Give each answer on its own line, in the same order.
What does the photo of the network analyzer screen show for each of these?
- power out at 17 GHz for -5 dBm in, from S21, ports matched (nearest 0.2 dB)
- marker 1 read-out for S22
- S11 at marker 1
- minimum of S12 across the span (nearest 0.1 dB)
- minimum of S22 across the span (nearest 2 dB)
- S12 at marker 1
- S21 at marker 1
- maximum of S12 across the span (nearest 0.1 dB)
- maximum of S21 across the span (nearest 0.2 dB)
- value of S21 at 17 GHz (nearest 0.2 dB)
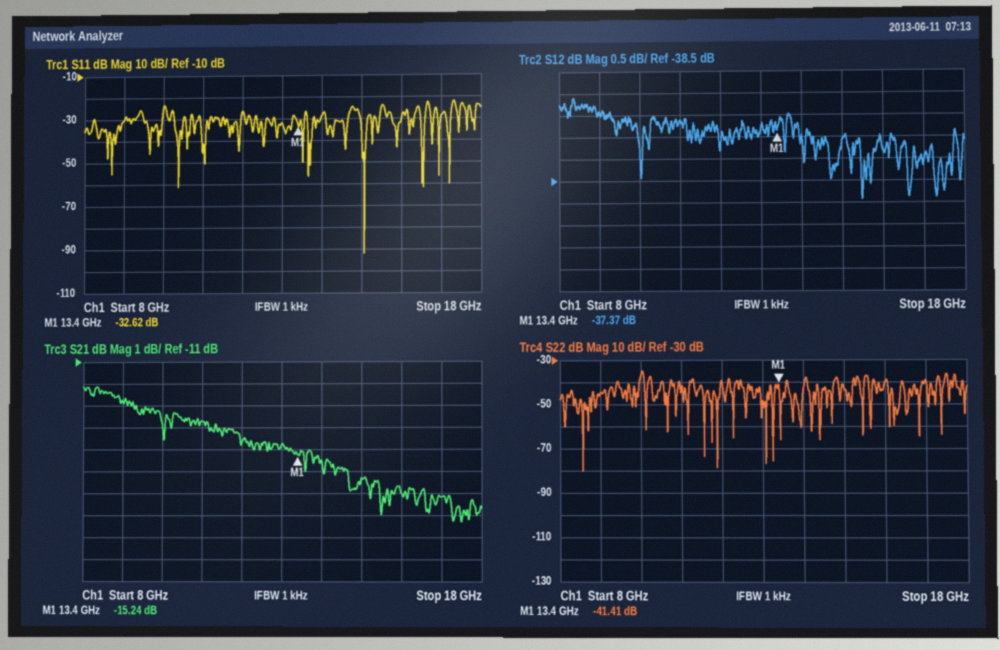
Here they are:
-22.2 dBm
-41.41 dB
-32.62 dB
-38.9 dB
-80 dB
-37.37 dB
-15.24 dB
-36.6 dB
-12.2 dB
-17.2 dB
